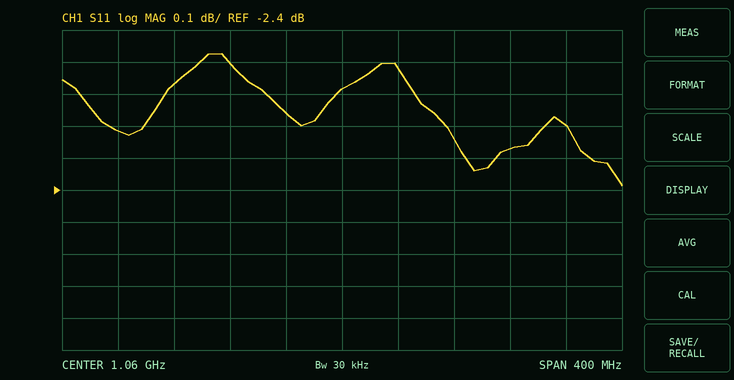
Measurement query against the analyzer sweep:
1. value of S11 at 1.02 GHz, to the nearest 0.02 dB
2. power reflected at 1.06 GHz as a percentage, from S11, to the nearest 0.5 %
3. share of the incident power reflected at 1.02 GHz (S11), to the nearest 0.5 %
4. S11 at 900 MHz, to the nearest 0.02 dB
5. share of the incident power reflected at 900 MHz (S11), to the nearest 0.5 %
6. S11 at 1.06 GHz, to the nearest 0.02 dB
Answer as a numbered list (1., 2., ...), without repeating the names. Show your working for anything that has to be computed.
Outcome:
1. -2.16 dB
2. 10^(-2.08/10) ≈ 61.9 %, so 62.0 % to the nearest 0.5 %
3. 10^(-2.16/10) ≈ 60.8 %, so 61.0 % to the nearest 0.5 %
4. -2.22 dB
5. 10^(-2.22/10) ≈ 60.0 %
6. -2.08 dB
